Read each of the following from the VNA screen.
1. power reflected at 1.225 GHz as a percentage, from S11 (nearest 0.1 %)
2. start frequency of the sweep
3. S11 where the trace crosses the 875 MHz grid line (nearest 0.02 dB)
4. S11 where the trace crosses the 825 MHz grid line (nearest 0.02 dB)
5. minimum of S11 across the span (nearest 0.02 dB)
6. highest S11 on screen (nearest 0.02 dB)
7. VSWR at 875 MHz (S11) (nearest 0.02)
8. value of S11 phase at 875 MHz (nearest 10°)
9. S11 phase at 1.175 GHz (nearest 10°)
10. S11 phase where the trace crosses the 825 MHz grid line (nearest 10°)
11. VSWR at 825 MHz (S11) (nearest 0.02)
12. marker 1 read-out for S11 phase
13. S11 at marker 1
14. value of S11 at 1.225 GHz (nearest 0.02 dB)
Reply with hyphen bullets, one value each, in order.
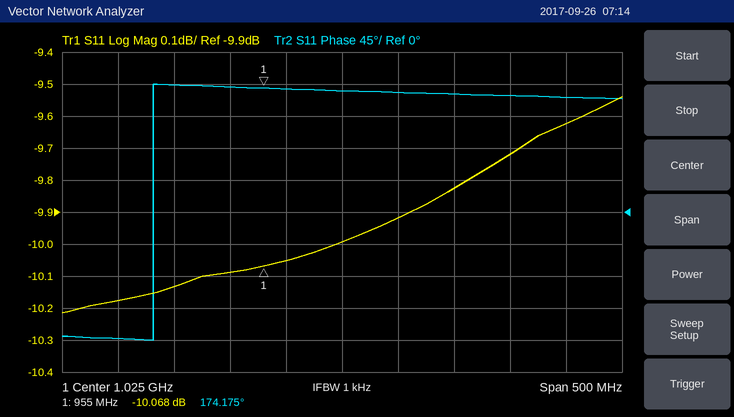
- 10.9 %
- 775 MHz
- -10.14 dB
- -10.18 dB
- -10.22 dB
- -9.54 dB
- 1.90
- 180°
- 160°
- -180°
- 1.90
- 174.175°
- -10.068 dB
- -9.62 dB
